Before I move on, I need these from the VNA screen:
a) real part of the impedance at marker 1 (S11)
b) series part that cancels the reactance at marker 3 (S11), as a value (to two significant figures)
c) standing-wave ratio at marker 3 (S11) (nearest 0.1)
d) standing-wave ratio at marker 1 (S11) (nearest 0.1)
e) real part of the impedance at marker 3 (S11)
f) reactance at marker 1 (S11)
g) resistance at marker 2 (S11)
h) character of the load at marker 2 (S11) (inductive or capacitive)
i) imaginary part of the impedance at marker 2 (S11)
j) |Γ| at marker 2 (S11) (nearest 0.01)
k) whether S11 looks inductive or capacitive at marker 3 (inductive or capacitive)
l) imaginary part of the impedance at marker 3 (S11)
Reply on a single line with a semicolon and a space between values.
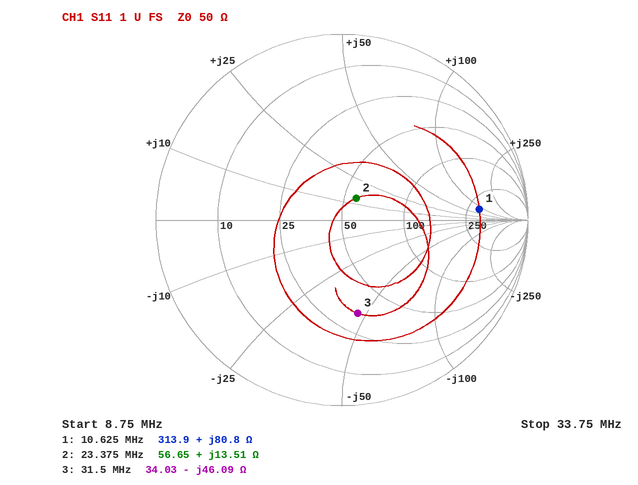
313.9 Ω; 230 nH; 3.1; 6.7; 34.03 Ω; +80.8 Ω; 56.65 Ω; inductive; +13.51 Ω; 0.14; capacitive; -46.09 Ω
